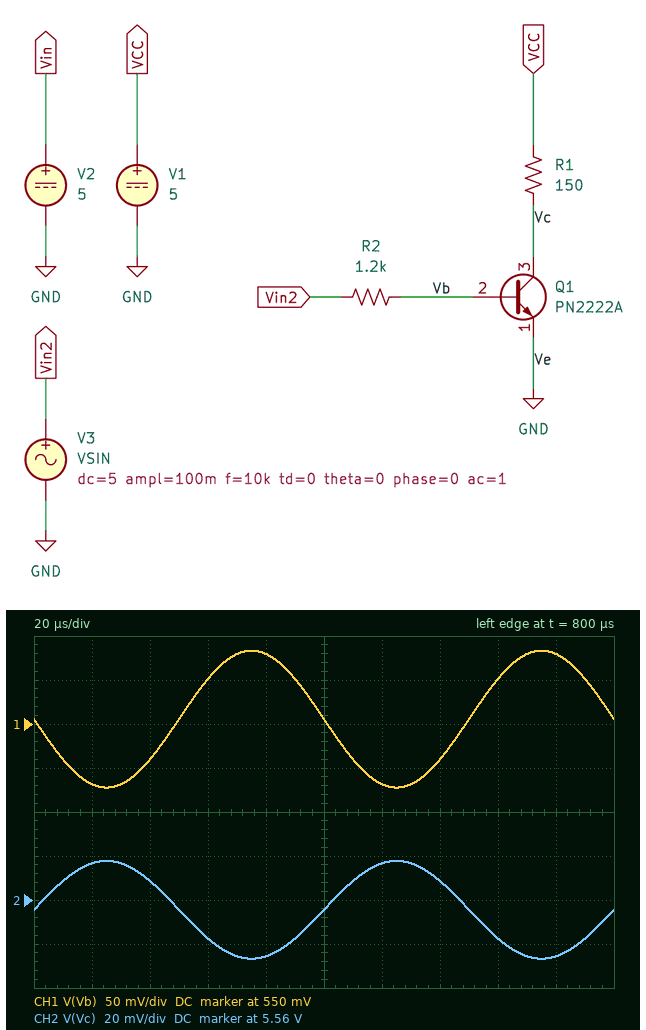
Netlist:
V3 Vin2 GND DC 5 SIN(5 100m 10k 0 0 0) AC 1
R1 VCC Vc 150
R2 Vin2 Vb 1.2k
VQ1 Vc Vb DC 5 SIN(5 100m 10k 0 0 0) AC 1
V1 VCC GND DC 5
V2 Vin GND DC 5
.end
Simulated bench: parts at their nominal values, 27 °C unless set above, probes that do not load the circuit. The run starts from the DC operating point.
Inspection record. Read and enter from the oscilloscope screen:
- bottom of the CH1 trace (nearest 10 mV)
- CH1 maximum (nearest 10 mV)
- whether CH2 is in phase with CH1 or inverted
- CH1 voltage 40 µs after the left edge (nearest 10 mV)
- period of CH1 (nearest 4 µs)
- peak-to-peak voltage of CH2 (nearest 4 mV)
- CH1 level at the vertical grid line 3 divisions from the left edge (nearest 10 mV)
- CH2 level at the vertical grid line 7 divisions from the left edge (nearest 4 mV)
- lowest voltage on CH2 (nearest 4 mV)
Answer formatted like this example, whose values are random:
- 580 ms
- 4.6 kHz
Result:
- 480 mV
- 630 mV
- inverted
- 510 mV
- 100 µs
- 44 mV
- 600 mV
- 5.568 V
- 5.532 V
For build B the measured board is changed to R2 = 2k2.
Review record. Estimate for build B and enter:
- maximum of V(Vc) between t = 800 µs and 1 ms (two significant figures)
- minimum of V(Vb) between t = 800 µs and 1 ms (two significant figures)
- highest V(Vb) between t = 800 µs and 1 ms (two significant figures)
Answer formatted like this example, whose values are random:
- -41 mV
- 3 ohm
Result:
- 5.3 V
- 230 mV
- 410 mV
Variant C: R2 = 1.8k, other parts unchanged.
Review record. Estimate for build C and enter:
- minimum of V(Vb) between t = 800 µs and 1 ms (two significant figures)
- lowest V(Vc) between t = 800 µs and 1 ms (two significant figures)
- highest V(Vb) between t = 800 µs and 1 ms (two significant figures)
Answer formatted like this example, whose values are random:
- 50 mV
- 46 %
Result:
- 300 mV
- 5.4 V
- 470 mV
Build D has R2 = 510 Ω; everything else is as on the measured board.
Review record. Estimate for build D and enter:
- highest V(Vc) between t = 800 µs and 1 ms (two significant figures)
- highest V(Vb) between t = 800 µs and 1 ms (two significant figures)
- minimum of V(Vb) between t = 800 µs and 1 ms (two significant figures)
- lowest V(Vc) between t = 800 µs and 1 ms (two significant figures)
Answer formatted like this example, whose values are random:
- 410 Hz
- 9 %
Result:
- 6.2 V
- 1.2 V
- 1.1 V
- 6.1 V
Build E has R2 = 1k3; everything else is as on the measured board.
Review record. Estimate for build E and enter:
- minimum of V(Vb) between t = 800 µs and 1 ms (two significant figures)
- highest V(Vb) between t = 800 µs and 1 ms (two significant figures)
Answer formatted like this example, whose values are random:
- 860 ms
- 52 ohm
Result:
- 440 mV
- 600 mV
